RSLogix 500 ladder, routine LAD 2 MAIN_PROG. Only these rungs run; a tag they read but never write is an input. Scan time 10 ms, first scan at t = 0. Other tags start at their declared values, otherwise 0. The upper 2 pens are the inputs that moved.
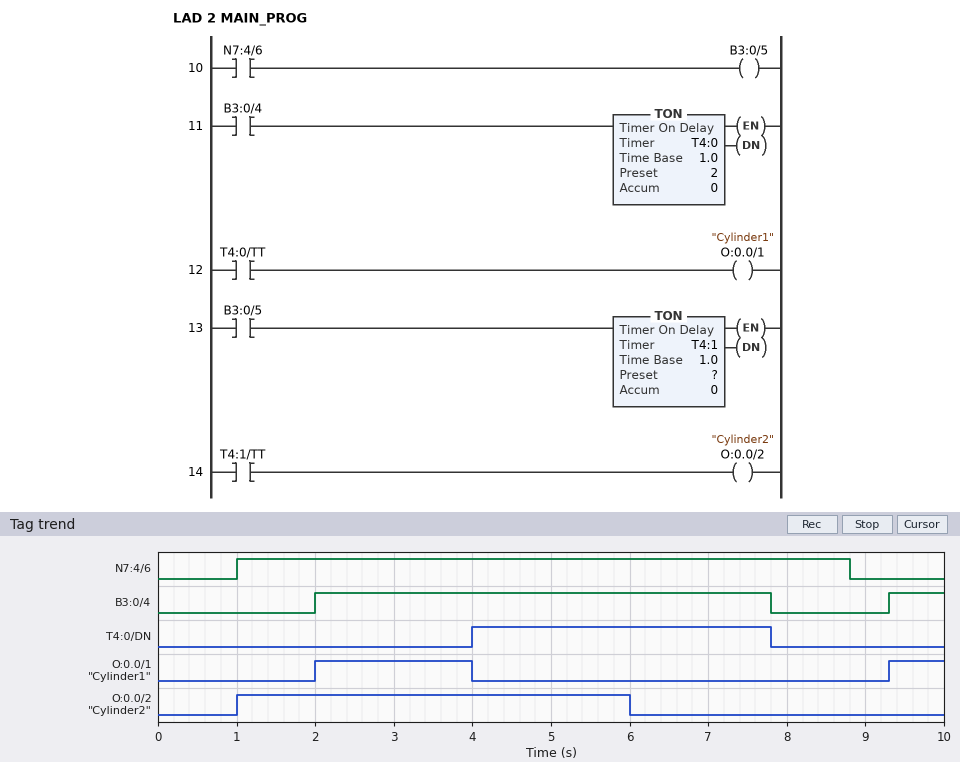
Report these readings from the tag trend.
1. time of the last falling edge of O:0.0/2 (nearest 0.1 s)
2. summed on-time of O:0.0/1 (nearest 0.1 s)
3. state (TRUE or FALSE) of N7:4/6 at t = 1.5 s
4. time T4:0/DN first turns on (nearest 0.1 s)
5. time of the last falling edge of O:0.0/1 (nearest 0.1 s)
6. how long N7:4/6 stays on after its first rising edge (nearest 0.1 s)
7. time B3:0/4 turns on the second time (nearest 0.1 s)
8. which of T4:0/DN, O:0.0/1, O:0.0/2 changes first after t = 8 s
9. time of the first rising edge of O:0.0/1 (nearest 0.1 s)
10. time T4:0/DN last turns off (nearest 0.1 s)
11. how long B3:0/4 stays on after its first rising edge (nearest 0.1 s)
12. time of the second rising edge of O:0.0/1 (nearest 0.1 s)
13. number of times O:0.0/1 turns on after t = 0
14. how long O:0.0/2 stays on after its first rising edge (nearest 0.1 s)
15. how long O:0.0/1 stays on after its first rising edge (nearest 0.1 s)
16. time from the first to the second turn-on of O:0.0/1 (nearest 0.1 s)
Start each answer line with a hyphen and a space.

- 6.0 s
- 2.7 s
- TRUE
- 4.0 s
- 4.0 s
- 7.8 s
- 9.3 s
- O:0.0/1
- 2.0 s
- 7.8 s
- 5.8 s
- 9.3 s
- 2
- 5.0 s
- 2.0 s
- 7.3 s
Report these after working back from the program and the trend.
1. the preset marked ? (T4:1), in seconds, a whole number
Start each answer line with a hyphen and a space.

- 5 s
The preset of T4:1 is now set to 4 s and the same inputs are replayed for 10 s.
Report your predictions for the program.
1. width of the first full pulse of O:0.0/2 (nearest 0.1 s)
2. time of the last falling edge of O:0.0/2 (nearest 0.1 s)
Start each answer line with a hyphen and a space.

- 4.0 s
- 5.0 s
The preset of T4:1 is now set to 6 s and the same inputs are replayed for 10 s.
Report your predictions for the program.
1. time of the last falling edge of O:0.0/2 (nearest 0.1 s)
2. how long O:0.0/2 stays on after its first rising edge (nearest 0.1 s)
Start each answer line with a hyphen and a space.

- 7.0 s
- 6.0 s
